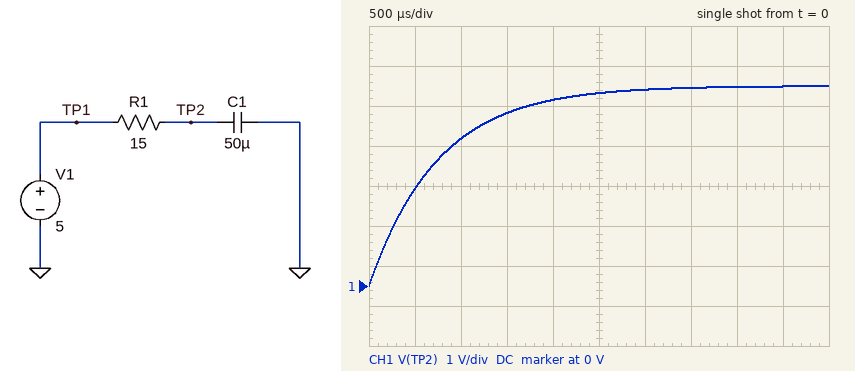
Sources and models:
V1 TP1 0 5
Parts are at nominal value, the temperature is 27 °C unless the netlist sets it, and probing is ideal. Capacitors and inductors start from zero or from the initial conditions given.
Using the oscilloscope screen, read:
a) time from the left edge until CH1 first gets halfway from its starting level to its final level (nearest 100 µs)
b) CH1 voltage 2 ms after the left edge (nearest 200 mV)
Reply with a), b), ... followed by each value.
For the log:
a) 500 µs
b) 4.6 V
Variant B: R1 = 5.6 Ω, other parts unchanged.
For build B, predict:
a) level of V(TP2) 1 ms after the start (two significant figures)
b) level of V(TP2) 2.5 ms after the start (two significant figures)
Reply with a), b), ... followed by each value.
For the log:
a) 4.9 V
b) 5.0 V
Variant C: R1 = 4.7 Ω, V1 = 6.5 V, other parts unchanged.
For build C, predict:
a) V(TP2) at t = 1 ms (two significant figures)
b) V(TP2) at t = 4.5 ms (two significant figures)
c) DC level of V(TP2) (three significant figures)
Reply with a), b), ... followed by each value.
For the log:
a) 6.4 V
b) 6.5 V
c) 6.50 V
